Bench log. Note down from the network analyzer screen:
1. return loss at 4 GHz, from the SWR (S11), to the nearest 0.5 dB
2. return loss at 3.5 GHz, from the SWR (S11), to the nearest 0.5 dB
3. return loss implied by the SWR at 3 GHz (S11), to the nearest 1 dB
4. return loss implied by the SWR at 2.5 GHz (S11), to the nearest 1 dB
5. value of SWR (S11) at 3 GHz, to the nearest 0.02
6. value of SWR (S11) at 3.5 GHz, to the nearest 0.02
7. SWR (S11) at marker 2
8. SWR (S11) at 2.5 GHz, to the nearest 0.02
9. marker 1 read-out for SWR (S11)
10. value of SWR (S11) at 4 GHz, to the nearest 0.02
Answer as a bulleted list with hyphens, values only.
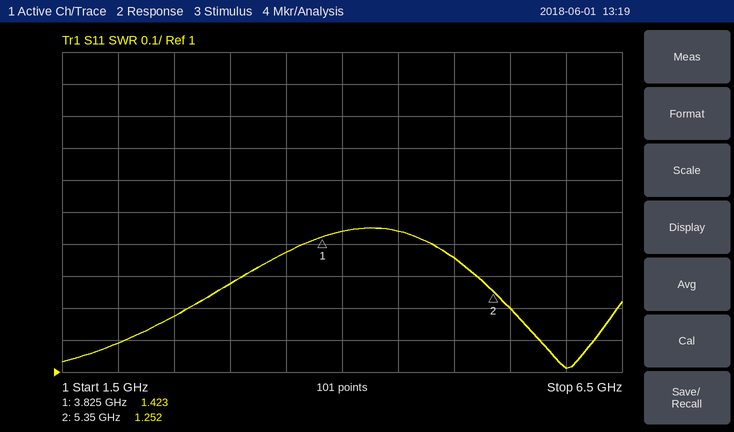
- 15.0 dB
- 16.0 dB
- 18 dB
- 22 dB
- 1.28
- 1.38
- 1.252
- 1.18
- 1.423
- 1.44
